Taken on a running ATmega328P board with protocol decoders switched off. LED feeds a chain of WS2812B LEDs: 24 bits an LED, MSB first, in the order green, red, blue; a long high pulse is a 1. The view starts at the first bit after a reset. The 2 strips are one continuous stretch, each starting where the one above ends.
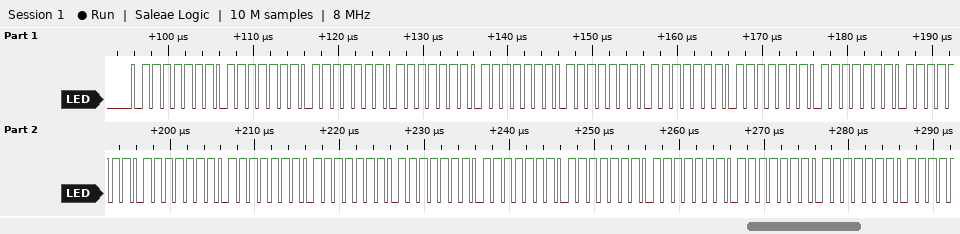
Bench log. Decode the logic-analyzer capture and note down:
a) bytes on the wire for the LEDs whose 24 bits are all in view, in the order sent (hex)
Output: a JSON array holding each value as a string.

["7F 7F 7F 7F 7F 7F 7F 7F 7F 7F 7F 7F 7F 7F 7F 7F 7F 7F"]
